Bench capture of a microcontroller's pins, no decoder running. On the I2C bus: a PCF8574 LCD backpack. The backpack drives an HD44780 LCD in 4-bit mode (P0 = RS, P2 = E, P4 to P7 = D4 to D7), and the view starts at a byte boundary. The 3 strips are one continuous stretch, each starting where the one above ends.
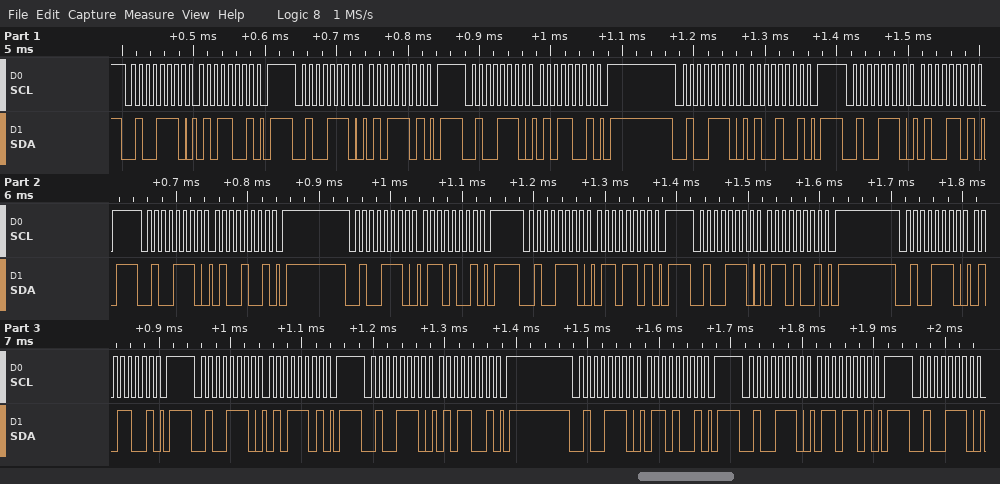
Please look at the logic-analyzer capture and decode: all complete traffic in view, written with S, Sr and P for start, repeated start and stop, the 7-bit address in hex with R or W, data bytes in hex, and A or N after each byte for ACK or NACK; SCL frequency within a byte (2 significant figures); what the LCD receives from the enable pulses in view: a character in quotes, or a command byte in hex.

S 27W A 59 A P S 27W A 5D A P S 27W A 59 A P S 27W A 49 A P S 27W A 4D A P S 27W A 49 A P S 27W A 69 A P S 27W A 6D A P S 27W A 69 A P S 27W A 59 A P S 27W A 5D A P S 27W A 59 A P S 27W A 69 A P S 27W A 6D A P S 27W A
100 kHz
'T' 'e'
